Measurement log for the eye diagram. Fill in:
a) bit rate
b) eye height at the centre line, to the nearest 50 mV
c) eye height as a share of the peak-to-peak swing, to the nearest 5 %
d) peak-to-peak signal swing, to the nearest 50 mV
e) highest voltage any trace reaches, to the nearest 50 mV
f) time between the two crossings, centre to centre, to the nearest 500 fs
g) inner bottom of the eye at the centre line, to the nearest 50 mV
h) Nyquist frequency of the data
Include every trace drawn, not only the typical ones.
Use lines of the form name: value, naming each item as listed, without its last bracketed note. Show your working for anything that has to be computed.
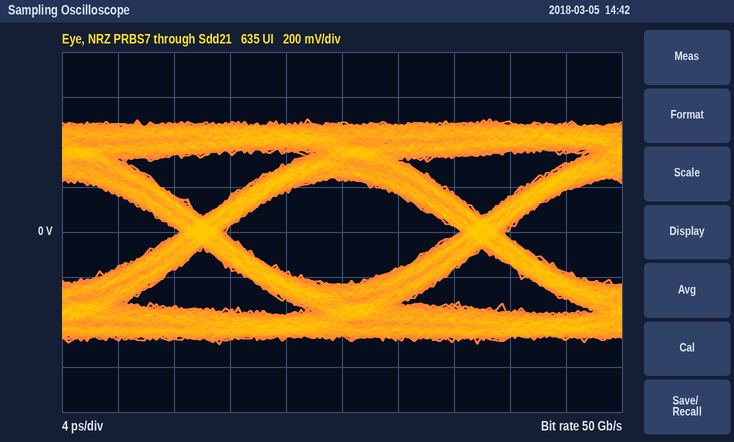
bit rate: 50 Gb/s
eye height at the centre line, to the nearest 50 mV: 450 mV
eye height as a share of the peak-to-peak swing, to the nearest 5 %: 450 mV / 1.00 V ≈ 45 %
peak-to-peak signal swing, to the nearest 50 mV: 1.00 V
highest voltage any trace reaches, to the nearest 50 mV: 500 mV
time between the two crossings, centre to centre, to the nearest 500 fs: 20.0 ps
inner bottom of the eye at the centre line, to the nearest 50 mV: -250 mV
Nyquist frequency of the data: 25 GHz
